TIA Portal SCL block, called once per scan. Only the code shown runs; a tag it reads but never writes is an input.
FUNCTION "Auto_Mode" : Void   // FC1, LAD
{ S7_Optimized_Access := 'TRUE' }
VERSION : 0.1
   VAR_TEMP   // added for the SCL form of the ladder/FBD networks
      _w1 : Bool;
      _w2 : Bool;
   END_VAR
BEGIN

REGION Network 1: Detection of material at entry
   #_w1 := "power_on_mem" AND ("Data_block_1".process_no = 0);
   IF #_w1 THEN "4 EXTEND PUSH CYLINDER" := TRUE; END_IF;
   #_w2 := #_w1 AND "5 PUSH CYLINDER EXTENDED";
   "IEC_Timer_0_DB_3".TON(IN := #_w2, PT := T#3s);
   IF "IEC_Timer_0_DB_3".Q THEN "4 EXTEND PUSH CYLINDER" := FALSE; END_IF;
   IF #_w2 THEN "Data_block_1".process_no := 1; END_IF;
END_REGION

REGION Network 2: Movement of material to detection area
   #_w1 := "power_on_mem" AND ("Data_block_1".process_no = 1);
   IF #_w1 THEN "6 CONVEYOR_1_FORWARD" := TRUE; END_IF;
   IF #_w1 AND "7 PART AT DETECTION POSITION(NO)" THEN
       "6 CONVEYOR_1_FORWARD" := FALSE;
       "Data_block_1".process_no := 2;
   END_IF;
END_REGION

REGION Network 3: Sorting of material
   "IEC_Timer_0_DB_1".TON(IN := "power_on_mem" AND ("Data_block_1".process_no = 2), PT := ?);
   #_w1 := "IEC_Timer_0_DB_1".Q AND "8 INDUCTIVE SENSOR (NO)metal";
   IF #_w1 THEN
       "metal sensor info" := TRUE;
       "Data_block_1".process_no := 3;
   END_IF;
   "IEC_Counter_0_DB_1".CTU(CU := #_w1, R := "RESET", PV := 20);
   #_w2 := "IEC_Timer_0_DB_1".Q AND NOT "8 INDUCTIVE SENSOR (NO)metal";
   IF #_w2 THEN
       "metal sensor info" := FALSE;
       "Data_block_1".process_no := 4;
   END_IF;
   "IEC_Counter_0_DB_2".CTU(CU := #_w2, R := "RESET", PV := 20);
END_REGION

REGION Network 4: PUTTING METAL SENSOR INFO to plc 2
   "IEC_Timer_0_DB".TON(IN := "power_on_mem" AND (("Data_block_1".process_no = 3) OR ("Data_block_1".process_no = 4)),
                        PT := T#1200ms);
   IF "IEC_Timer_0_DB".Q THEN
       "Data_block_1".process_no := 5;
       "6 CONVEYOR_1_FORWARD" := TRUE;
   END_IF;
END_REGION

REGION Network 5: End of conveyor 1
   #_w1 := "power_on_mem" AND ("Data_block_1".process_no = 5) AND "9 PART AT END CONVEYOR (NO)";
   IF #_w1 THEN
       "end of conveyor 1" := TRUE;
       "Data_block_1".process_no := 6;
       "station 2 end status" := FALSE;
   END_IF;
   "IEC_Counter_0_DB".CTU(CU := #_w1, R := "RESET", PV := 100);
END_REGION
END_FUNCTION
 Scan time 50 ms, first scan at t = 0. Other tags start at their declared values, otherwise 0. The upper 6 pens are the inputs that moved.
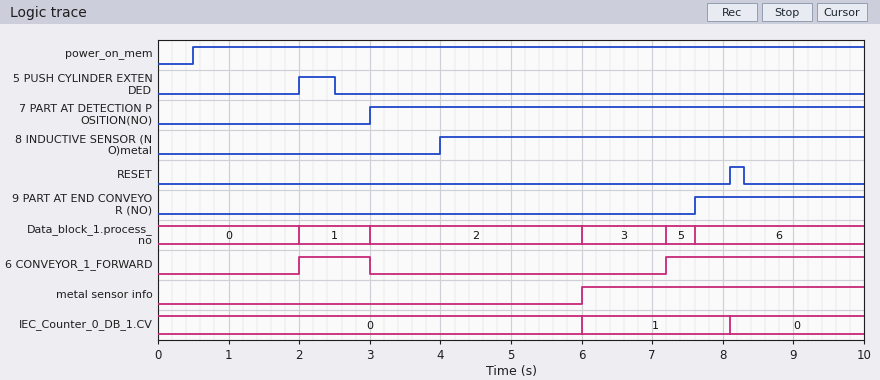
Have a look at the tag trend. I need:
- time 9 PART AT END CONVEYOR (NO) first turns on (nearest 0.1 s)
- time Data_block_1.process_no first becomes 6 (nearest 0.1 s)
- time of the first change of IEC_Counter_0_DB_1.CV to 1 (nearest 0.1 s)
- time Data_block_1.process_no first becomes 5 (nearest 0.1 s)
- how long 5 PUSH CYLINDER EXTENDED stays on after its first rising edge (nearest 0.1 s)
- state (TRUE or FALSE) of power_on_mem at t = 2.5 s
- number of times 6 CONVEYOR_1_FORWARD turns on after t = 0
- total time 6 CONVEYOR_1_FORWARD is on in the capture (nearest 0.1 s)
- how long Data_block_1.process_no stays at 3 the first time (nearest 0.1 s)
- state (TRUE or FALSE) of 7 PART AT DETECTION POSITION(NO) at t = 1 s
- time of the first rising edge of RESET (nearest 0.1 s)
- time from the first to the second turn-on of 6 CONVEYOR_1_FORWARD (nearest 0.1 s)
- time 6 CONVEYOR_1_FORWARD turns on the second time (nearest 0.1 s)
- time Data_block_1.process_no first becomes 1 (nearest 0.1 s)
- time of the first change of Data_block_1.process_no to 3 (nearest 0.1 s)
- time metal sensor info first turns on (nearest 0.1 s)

7.6 s
7.6 s
6.0 s
7.2 s
0.5 s
TRUE
2
3.8 s
1.2 s
FALSE
8.1 s
5.2 s
7.2 s
2.0 s
6.0 s
6.0 s
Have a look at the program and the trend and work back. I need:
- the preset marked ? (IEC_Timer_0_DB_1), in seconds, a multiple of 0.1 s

3.0 s
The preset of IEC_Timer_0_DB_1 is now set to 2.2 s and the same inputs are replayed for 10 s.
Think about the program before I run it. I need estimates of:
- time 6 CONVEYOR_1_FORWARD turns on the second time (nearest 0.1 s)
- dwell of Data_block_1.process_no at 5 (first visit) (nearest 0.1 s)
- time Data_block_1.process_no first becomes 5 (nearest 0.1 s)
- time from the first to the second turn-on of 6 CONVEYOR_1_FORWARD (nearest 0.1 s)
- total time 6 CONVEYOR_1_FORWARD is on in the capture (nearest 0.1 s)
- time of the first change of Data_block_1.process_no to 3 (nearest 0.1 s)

6.4 s
1.2 s
6.4 s
4.4 s
4.6 s
5.2 s
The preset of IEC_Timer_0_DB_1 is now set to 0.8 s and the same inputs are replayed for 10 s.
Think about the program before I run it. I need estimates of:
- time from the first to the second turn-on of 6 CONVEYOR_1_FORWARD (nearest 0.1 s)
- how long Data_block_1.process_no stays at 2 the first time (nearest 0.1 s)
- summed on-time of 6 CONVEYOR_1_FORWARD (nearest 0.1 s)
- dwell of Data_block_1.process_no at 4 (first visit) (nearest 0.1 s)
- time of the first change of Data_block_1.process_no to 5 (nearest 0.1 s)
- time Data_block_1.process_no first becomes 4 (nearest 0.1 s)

3.0 s
0.8 s
6.0 s
1.2 s
5.0 s
3.8 s
